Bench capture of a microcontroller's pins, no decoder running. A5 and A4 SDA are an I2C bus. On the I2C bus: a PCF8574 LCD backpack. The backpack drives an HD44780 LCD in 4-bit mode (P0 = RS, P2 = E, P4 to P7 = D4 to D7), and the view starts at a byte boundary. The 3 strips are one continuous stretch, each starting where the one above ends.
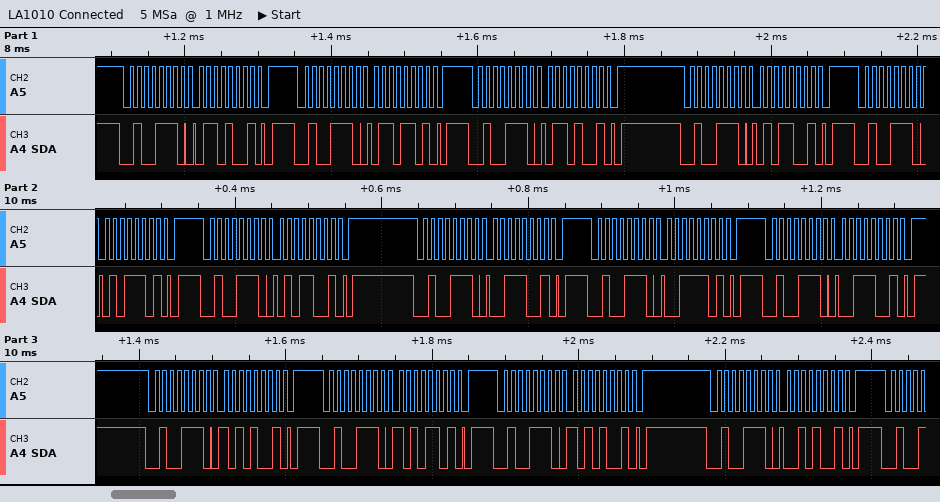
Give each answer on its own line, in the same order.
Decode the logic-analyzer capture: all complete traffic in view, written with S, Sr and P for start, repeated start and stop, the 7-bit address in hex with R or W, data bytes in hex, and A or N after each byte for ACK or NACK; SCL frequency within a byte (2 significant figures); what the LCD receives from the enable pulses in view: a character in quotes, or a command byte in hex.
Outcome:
S 27W A 69 A P S 27W A 6D A P S 27W A 69 A P S 27W A 59 A P S 27W A 5D A P S 27W A 59 A P S 27W A 39 A P S 27W A 3D A P S 27W A 39 A P S 27W A A9 A P S 27W A AD A P S 27W A A9 A P S 27W A 29 A P
100 kHz
'e' ':'
